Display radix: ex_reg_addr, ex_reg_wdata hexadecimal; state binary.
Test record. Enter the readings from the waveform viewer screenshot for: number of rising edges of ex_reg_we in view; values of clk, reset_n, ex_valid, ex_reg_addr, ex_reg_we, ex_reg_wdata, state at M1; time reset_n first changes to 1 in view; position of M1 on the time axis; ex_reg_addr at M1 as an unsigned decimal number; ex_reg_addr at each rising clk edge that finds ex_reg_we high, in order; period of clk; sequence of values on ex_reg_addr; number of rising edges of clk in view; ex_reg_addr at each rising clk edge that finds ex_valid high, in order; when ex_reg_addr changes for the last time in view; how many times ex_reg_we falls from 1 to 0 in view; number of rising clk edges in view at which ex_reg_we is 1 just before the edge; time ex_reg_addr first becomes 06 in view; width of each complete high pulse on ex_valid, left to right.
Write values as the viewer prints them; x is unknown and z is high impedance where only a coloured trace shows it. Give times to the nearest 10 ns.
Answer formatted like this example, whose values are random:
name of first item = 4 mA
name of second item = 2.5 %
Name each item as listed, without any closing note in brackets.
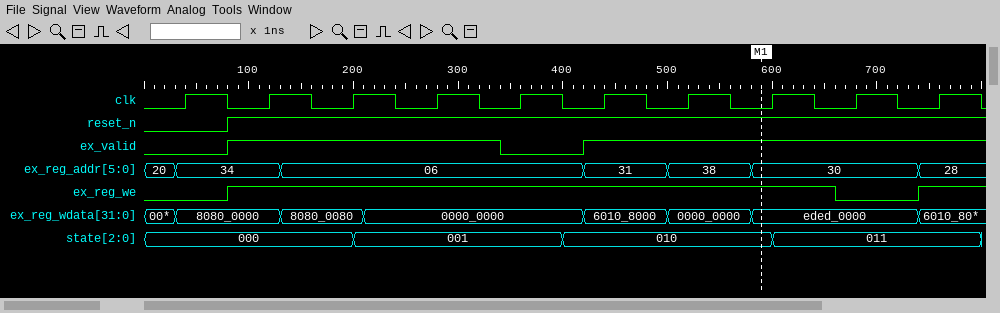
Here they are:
number of rising edges of ex_reg_we in view = 2
values of clk, reset_n, ex_valid, ex_reg_addr, ex_reg_we, ex_reg_wdata, state at M1 = clk=0, reset_n=1, ex_valid=1, ex_reg_addr=30, ex_reg_we=1, ex_reg_wdata=eded_0000, state=010
time reset_n first changes to 1 in view = 80 ns
position of M1 on the time axis = 590 ns
ex_reg_addr at M1 as an unsigned decimal number = 48
ex_reg_addr at each rising clk edge that finds ex_reg_we high, in order = 34, 06, 06, 06, 31, 38, 30, 28
period of clk = 80 ns
sequence of values on ex_reg_addr = 20, 34, 06, 31, 38, 30, 28
number of rising edges of clk in view = 10
ex_reg_addr at each rising clk edge that finds ex_valid high, in order = 34, 06, 06, 31, 38, 30, 30, 28
when ex_reg_addr changes for the last time in view = 740 ns
how many times ex_reg_we falls from 1 to 0 in view = 1
number of rising clk edges in view at which ex_reg_we is 1 just before the edge = 8
time ex_reg_addr first becomes 06 in view = 130 ns
width of each complete high pulse on ex_valid, left to right = 260 ns
